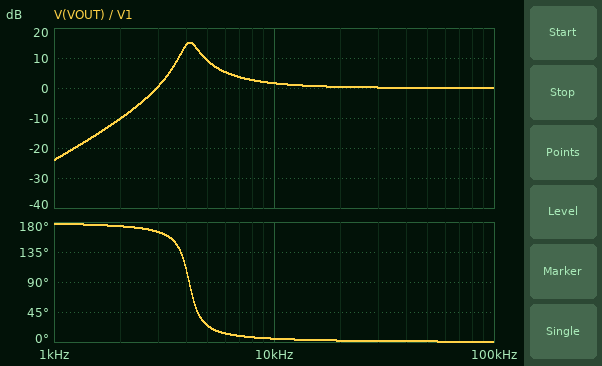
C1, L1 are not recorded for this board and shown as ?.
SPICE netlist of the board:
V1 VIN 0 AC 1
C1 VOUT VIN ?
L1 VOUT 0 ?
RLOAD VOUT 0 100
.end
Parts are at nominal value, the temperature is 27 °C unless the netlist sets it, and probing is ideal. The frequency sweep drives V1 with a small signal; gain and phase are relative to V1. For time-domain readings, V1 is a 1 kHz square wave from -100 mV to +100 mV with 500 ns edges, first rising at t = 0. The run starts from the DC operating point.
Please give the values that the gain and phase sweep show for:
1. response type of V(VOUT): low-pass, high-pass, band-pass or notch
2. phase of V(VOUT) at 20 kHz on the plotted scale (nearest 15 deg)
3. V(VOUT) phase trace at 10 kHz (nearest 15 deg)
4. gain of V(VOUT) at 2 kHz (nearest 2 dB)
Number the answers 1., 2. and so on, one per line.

1. high-pass
2. 0 deg
3. 0 deg
4. -10 dB
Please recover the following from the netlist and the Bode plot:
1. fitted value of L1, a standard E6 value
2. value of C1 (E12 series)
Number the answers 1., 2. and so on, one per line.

1. 680 µH
2. 2.2 µF
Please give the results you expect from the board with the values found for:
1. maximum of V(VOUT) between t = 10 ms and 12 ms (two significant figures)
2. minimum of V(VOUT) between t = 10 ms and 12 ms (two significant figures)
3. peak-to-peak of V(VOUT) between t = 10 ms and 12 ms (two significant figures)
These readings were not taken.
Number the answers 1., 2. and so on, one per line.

1. 150 mV
2. -150 mV
3. 310 mV
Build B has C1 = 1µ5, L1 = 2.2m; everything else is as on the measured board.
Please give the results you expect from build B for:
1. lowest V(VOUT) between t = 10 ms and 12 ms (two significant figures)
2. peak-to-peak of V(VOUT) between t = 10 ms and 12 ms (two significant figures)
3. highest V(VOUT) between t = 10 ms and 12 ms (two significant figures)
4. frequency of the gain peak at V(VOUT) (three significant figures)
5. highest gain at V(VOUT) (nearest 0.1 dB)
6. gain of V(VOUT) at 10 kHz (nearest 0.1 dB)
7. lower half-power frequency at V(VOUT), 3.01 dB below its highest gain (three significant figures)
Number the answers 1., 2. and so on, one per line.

1. -230 mV
2. 460 mV
3. 230 mV
4. 2.88 kHz
5. 8.5 dB
6. 0.6 dB
7. 2.43 kHz
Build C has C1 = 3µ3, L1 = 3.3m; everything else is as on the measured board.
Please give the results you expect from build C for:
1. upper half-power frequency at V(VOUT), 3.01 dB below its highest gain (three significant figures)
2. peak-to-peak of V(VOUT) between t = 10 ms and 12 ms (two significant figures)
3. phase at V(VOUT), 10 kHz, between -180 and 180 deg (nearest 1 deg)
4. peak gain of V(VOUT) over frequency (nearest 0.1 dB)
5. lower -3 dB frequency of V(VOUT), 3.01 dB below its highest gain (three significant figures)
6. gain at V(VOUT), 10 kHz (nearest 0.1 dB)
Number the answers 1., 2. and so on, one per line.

1. 1.91 kHz
2. 300 mV
3. 3 deg
4. 10.1 dB
5. 1.36 kHz
6. 0.2 dB
